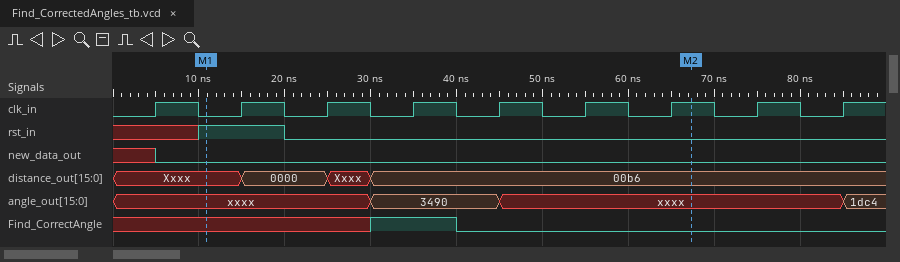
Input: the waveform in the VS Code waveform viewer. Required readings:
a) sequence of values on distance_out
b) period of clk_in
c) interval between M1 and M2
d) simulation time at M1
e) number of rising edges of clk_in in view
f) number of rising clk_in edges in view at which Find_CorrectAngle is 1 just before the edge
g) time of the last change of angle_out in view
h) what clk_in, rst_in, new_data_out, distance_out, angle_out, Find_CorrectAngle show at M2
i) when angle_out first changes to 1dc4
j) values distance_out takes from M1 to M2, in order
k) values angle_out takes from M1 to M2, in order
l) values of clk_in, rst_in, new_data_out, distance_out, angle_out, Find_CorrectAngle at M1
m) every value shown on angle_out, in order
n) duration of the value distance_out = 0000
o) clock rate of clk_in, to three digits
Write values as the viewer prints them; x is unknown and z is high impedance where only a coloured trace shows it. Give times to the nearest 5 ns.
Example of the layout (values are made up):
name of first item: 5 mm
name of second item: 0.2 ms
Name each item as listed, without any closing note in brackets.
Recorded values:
sequence of values on distance_out: Xxxx, 0000, Xxxx, 00b6
period of clk_in: 10 ns
interval between M1 and M2: 55 ns
simulation time at M1: 10 ns
number of rising edges of clk_in in view: 9
number of rising clk_in edges in view at which Find_CorrectAngle is 1 just before the edge: 1
time of the last change of angle_out in view: 85 ns
what clk_in, rst_in, new_data_out, distance_out, angle_out, Find_CorrectAngle show at M2: clk_in=1, rst_in=0, new_data_out=0, distance_out=00b6, angle_out=xxxx, Find_CorrectAngle=0
when angle_out first changes to 1dc4: 85 ns
values distance_out takes from M1 to M2, in order: Xxxx, 0000, Xxxx, 00b6
values angle_out takes from M1 to M2, in order: xxxx, 3490, xxxx
values of clk_in, rst_in, new_data_out, distance_out, angle_out, Find_CorrectAngle at M1: clk_in=0, rst_in=1, new_data_out=0, distance_out=Xxxx, angle_out=xxxx, Find_CorrectAngle=x
every value shown on angle_out, in order: xxxx, 3490, xxxx, 1dc4
duration of the value distance_out = 0000: 10 ns
clock rate of clk_in, to three digits: 100 MHz
